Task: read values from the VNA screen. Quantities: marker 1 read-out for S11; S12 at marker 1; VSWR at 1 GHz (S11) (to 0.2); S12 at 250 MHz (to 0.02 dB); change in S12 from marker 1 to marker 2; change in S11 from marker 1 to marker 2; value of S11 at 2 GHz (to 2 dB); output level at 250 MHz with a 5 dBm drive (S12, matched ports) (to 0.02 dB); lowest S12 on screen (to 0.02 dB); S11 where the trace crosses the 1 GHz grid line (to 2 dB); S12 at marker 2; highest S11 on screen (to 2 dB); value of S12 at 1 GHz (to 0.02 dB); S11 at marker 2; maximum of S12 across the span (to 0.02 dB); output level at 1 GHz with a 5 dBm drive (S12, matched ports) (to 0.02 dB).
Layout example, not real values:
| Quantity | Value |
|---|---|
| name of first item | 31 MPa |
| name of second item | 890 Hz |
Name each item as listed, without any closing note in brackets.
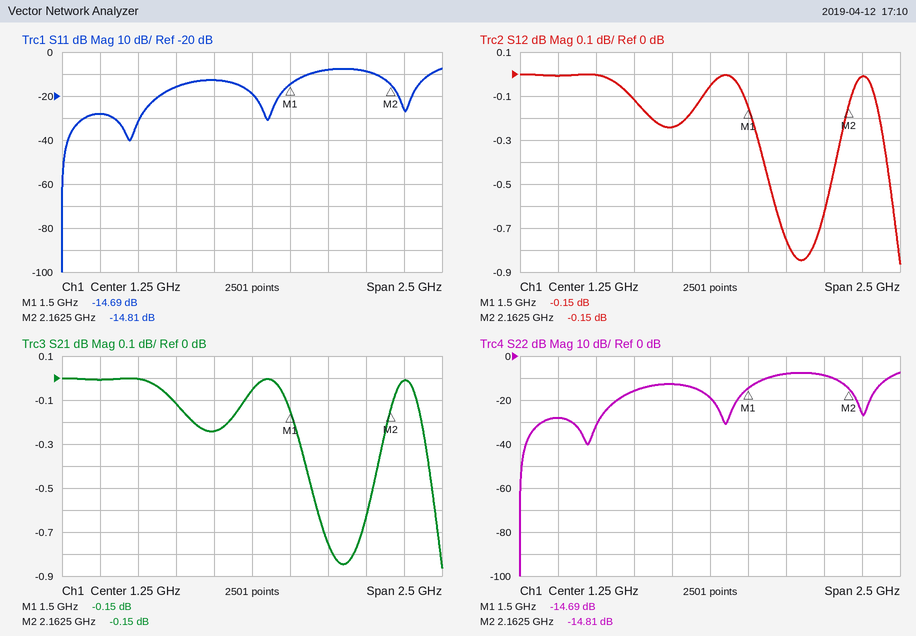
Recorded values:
| Quantity | Value |
|---|---|
| marker 1 read-out for S11 | -14.69 dB |
| S12 at marker 1 | -0.15 dB |
| VSWR at 1 GHz (S11) | 1.6 |
| S12 at 250 MHz | 0.00 dB |
| change in S12 from marker 1 to marker 2 | 0.00 dB |
| change in S11 from marker 1 to marker 2 | -0.12 dB |
| value of S11 at 2 GHz | -8 dB |
| output level at 250 MHz with a 5 dBm drive (S12, matched ports) | 5.00 dBm |
| lowest S12 on screen | -0.86 dB |
| S11 where the trace crosses the 1 GHz grid line | -12 dB |
| S12 at marker 2 | -0.15 dB |
| highest S11 on screen | -8 dB |
| value of S12 at 1 GHz | -0.24 dB |
| S11 at marker 2 | -14.81 dB |
| maximum of S12 across the span | 0.00 dB |
| output level at 1 GHz with a 5 dBm drive (S12, matched ports) | 4.76 dBm |
